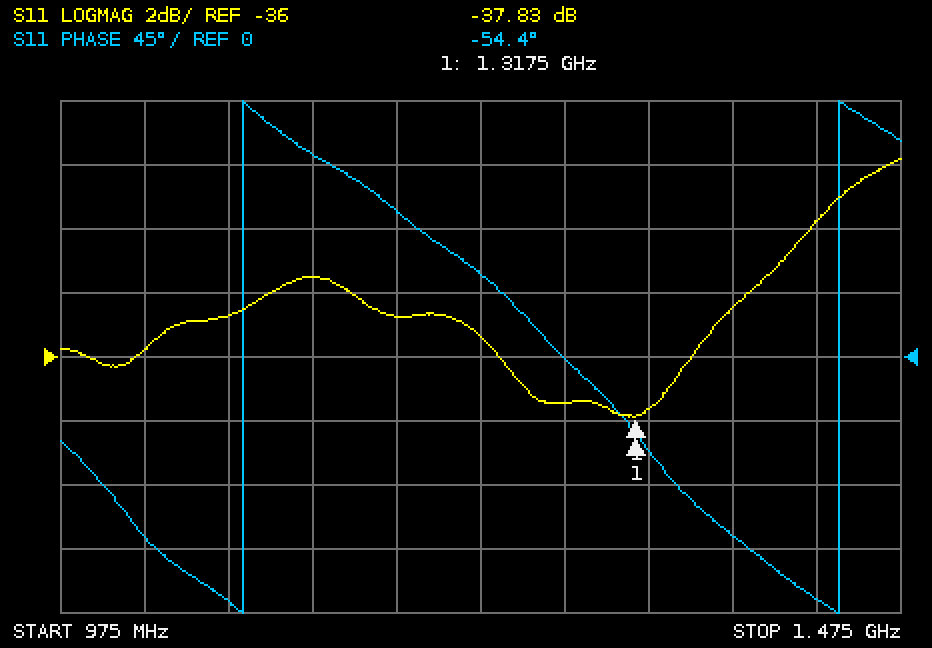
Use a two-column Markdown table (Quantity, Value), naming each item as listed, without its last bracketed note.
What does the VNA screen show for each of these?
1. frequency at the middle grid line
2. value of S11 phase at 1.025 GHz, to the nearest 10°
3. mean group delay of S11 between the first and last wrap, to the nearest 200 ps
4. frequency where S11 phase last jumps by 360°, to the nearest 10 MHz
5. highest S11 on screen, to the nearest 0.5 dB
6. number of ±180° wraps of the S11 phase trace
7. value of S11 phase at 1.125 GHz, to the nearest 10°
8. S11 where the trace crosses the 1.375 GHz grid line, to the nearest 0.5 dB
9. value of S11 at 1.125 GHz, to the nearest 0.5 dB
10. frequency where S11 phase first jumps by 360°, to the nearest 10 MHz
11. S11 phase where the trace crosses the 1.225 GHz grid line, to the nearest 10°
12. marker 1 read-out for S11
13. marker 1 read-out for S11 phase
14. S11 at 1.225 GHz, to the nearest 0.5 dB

| Quantity | Value |
|---|---|
| frequency at the middle grid line | 1.225 GHz |
| value of S11 phase at 1.025 GHz, to the nearest 10° | -130° |
| mean group delay of S11 between the first and last wrap, to the nearest 200 ps | 2.8 ns |
| frequency where S11 phase last jumps by 360°, to the nearest 10 MHz | 1.44 GHz |
| highest S11 on screen, to the nearest 0.5 dB | -30.0 dB |
| number of ±180° wraps of the S11 phase trace | 2 |
| value of S11 phase at 1.125 GHz, to the nearest 10° | 140° |
| S11 where the trace crosses the 1.375 GHz grid line, to the nearest 0.5 dB | -34.5 dB |
| value of S11 at 1.125 GHz, to the nearest 0.5 dB | -33.5 dB |
| frequency where S11 phase first jumps by 360°, to the nearest 10 MHz | 1.08 GHz |
| S11 phase where the trace crosses the 1.225 GHz grid line, to the nearest 10° | 60° |
| marker 1 read-out for S11 | -37.83 dB |
| marker 1 read-out for S11 phase | -54.4° |
| S11 at 1.225 GHz, to the nearest 0.5 dB | -35.5 dB |
